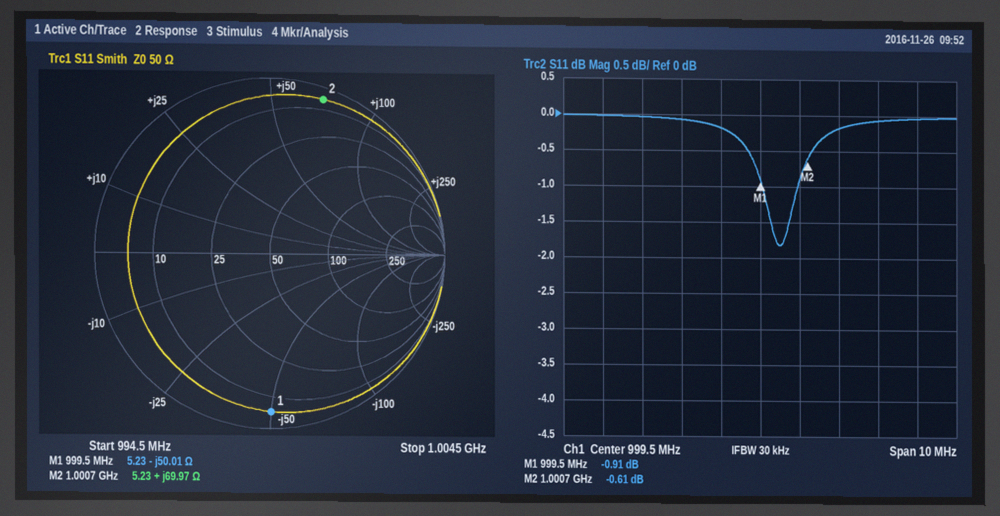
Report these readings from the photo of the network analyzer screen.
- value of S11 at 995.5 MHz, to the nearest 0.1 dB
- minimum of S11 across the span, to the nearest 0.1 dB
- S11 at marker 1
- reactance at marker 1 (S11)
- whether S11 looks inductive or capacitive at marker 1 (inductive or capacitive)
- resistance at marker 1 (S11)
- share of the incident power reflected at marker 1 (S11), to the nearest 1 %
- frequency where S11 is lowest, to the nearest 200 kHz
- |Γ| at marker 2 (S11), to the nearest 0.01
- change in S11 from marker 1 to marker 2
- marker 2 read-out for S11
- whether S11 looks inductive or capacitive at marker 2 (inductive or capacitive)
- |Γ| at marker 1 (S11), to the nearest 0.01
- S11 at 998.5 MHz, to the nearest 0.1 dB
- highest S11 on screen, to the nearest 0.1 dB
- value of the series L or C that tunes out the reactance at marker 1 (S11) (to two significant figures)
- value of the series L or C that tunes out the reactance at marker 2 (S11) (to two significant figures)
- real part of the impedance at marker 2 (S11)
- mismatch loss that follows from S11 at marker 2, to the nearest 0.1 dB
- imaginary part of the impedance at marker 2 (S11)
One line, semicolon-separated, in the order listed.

0.0 dB; -1.8 dB; -0.91 dB; -50.01 Ω; capacitive; 5.23 Ω; 81 %; 1.0000 GHz; 0.93; 0.30 dB; -0.61 dB; inductive; 0.90; -0.2 dB; 0.0 dB; 8.0 nH; 2.3 pF; 5.23 Ω; 8.8 dB; +69.97 Ω
